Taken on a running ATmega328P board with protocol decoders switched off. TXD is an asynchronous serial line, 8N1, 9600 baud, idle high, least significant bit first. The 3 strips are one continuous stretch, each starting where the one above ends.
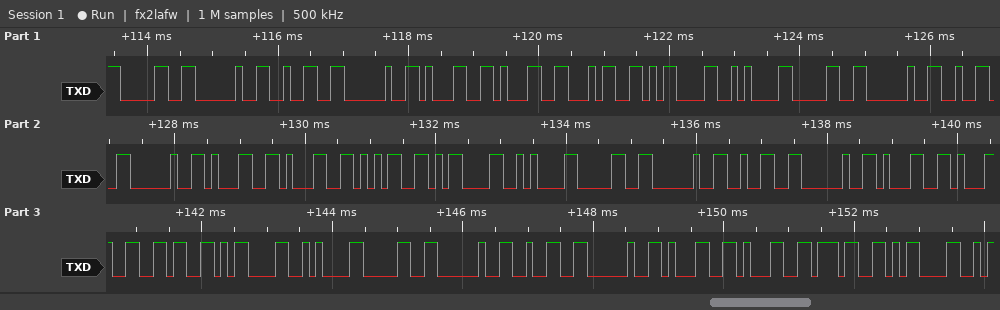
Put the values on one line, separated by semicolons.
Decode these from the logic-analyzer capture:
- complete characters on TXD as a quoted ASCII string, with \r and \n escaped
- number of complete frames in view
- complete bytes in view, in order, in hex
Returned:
"0 2 114\r\n0 2 115\r\n0 2 116\r\n0 2 117\r"; 35; 30 20 32 20 31 31 34 0D 0A 30 20 32 20 31 31 35 0D 0A 30 20 32 20 31 31 36 0D 0A 30 20 32 20 31 31 37 0D
